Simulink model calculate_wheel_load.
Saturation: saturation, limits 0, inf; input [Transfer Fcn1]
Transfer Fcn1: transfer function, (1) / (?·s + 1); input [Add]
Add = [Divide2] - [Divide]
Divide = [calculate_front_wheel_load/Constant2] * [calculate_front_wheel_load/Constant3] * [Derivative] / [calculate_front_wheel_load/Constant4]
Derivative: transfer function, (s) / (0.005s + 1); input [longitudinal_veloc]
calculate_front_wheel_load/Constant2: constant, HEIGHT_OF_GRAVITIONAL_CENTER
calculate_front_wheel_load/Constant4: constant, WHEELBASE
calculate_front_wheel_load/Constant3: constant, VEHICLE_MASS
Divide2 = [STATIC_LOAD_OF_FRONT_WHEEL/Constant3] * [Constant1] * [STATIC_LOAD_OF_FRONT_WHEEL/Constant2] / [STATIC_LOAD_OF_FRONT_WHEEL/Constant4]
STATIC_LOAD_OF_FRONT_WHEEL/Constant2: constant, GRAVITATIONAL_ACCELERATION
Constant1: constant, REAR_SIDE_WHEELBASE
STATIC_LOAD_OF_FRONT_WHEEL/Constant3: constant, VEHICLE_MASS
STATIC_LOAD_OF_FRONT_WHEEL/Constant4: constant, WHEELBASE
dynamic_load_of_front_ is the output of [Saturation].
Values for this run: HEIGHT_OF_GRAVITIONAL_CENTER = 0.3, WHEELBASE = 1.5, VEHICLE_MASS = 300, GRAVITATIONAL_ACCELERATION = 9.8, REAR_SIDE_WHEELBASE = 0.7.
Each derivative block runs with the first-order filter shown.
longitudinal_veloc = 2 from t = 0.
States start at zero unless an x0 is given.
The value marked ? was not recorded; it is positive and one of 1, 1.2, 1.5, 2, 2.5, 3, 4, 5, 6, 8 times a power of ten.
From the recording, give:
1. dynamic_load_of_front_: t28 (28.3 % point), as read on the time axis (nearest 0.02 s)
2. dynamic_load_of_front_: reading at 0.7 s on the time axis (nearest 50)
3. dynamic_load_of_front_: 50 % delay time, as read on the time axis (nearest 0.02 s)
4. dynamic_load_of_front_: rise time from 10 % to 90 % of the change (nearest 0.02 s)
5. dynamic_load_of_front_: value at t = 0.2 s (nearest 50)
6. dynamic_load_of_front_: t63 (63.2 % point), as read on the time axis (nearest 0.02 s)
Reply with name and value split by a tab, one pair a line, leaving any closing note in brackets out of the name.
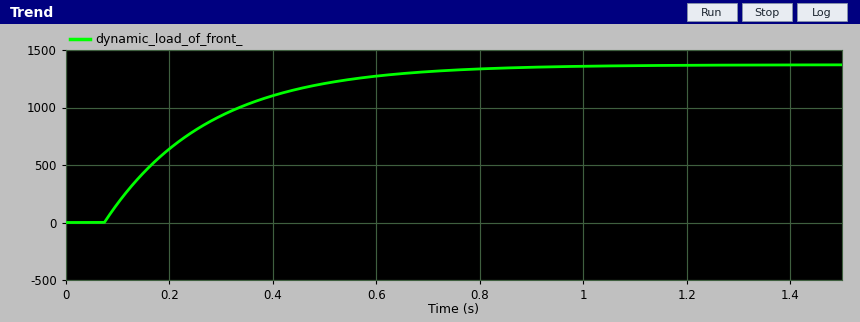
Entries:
dynamic_load_of_front_: t28 (28.3 % point), as read on the time axis	0.14 s
dynamic_load_of_front_: reading at 0.7 s on the time axis	1300
dynamic_load_of_front_: 50 % delay time, as read on the time axis	0.22 s
dynamic_load_of_front_: rise time from 10 % to 90 % of the change	0.44 s
dynamic_load_of_front_: value at t = 0.2 s	650
dynamic_load_of_front_: t63 (63.2 % point), as read on the time axis	0.28 s
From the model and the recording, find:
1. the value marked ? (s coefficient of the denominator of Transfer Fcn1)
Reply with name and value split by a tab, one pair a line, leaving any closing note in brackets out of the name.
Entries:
the value marked ?	0.2
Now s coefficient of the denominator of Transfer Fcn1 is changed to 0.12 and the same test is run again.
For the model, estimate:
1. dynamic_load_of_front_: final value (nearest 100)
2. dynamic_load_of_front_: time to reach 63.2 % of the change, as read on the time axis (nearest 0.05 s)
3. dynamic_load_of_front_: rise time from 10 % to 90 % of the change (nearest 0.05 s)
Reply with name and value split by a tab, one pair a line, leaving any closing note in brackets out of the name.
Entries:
dynamic_load_of_front_: final value	1400
dynamic_load_of_front_: time to reach 63.2 % of the change, as read on the time axis	0.20 s
dynamic_load_of_front_: rise time from 10 % to 90 % of the change	0.25 s
